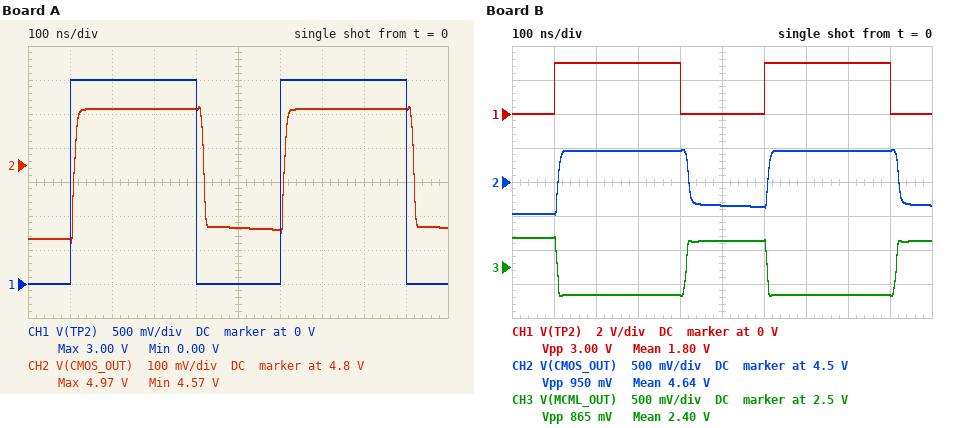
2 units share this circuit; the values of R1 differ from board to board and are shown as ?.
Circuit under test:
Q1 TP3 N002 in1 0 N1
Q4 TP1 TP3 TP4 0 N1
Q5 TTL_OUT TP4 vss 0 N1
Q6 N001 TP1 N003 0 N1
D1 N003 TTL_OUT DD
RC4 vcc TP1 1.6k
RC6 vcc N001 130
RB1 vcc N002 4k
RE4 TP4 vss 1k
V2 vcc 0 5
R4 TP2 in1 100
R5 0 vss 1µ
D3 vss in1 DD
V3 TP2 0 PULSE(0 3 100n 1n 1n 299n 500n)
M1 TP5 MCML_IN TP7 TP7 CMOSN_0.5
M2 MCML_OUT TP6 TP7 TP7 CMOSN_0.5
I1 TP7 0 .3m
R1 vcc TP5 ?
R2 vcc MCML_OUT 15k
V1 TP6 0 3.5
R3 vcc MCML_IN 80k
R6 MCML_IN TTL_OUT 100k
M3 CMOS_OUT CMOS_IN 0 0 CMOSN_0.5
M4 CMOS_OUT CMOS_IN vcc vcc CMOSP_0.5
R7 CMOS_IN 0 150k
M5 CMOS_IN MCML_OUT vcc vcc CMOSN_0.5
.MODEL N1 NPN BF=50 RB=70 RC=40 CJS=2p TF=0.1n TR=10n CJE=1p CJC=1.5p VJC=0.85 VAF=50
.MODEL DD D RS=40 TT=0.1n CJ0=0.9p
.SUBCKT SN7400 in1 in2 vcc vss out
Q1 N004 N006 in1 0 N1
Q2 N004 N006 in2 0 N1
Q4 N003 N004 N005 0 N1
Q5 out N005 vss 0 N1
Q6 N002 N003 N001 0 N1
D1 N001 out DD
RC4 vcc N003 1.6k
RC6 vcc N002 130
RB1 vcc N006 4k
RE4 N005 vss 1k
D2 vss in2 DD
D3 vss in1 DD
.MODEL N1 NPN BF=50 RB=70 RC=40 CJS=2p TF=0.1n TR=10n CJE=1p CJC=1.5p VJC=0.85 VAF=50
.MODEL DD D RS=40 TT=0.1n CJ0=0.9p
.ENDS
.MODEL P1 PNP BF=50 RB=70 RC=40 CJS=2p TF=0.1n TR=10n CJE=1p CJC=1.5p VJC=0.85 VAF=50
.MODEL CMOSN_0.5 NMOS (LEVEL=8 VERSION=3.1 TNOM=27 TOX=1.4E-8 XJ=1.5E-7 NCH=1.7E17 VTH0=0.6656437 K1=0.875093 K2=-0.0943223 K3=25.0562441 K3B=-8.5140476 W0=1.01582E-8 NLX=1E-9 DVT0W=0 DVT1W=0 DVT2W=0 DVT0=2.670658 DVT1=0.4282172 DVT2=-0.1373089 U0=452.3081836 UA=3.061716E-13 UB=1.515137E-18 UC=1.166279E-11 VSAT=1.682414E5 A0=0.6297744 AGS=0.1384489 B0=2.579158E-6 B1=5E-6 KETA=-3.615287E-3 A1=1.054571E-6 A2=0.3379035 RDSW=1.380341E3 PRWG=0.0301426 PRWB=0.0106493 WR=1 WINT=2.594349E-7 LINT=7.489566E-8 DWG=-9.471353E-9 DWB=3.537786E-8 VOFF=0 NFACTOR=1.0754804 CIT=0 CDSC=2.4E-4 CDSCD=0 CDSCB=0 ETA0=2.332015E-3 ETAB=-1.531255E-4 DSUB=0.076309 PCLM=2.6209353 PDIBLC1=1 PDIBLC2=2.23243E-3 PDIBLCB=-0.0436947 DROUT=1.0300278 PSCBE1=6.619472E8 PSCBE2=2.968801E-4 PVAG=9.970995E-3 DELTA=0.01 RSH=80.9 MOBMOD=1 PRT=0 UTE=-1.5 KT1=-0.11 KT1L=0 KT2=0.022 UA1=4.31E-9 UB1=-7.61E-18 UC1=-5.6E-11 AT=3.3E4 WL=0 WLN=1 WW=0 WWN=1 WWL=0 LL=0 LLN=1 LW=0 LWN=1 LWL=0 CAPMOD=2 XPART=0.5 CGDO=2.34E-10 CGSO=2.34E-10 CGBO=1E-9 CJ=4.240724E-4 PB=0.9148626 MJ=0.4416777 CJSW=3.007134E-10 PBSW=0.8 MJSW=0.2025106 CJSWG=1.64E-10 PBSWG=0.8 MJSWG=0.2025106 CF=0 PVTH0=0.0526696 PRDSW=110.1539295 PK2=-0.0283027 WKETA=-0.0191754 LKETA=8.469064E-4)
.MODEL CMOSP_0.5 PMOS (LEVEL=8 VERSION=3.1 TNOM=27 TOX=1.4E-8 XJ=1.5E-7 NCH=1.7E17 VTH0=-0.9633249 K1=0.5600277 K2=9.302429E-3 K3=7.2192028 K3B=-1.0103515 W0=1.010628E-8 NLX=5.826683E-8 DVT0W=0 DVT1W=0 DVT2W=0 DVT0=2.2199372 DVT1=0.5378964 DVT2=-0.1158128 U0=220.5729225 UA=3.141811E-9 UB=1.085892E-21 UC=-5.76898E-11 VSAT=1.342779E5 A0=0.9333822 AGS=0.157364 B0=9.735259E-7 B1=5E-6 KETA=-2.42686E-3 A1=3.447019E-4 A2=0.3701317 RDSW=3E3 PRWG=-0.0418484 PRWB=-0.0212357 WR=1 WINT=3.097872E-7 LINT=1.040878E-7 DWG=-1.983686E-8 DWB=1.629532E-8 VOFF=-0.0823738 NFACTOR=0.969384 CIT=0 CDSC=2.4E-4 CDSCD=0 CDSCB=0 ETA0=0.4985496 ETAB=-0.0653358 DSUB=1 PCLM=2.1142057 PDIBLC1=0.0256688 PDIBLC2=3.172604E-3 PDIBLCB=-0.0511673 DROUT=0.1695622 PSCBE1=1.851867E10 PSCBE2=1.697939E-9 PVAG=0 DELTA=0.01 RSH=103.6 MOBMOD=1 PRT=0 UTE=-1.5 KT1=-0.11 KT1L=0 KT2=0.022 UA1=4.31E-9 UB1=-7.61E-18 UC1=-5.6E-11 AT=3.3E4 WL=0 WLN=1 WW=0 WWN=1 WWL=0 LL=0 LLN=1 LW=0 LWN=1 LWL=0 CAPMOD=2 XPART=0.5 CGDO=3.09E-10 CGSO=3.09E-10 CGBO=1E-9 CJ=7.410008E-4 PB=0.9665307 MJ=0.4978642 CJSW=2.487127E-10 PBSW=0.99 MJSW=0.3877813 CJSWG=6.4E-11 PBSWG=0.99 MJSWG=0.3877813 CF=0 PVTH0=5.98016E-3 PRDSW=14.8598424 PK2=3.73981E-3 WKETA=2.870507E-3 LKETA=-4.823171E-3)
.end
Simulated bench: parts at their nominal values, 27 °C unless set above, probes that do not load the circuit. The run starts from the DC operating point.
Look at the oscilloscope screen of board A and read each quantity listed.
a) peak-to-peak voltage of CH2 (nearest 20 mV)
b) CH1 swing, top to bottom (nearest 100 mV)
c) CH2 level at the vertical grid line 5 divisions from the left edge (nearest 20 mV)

400 mV
3.0 V
4.62 V
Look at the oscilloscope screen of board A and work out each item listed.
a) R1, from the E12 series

27 kΩ
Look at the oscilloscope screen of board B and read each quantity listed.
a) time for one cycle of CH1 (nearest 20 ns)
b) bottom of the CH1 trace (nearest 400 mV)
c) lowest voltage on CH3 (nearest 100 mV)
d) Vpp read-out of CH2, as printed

500 ns
0 V
2.1 V
950 mV
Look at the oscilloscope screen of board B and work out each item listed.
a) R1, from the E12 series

22 kΩ
